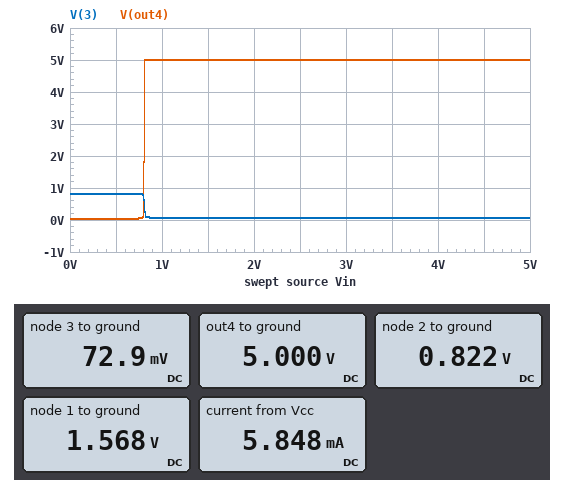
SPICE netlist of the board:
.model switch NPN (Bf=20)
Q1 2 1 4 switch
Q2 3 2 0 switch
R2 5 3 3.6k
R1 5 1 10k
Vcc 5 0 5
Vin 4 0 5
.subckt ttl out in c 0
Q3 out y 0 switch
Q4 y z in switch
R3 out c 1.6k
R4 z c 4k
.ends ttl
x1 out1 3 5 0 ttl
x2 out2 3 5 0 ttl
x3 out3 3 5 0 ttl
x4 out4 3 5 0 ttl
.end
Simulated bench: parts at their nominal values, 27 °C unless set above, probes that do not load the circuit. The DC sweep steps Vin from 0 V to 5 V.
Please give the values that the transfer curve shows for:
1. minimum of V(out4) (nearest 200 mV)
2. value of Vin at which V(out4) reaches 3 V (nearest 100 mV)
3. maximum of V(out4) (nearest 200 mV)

0 V
800 mV
5.0 V
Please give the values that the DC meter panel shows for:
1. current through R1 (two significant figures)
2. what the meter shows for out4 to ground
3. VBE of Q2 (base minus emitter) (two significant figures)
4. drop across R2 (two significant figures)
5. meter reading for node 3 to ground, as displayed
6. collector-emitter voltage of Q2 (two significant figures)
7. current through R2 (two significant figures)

340 µA
5.000 V
820 mV
4.9 V
72.9 mV
73 mV
1.4 mA
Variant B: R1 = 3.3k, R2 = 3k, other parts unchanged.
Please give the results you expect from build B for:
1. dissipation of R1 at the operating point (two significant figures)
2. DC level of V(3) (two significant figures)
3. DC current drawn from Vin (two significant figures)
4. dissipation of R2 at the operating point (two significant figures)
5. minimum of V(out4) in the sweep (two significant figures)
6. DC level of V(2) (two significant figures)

3.5 mW
45 mV
1.0 mA
8.2 mW
43 mV
830 mV
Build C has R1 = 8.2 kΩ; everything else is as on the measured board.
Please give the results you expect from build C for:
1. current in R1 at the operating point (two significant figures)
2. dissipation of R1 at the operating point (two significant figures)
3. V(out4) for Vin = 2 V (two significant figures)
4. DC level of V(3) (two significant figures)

420 µA
1.4 mW
5.0 V
66 mV
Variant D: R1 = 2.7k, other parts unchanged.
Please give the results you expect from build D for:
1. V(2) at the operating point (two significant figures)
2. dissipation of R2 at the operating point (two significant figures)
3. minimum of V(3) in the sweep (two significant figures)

830 mV
6.8 mW
40 mV
